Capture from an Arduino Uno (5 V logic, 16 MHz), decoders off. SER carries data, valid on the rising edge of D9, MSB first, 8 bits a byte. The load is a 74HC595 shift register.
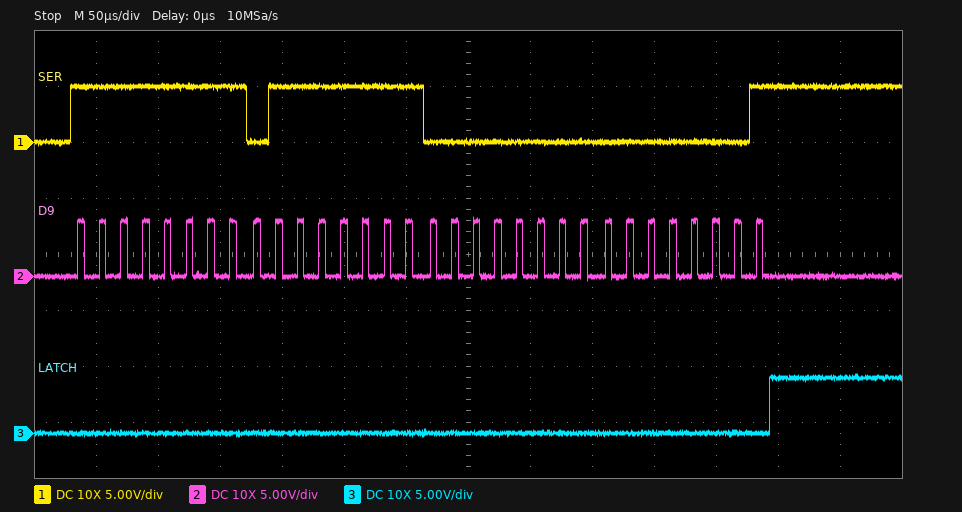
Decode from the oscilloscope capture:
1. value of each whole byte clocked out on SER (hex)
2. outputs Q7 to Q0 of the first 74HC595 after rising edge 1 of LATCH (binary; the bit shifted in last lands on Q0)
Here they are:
FF 7F 00 01
00000001
